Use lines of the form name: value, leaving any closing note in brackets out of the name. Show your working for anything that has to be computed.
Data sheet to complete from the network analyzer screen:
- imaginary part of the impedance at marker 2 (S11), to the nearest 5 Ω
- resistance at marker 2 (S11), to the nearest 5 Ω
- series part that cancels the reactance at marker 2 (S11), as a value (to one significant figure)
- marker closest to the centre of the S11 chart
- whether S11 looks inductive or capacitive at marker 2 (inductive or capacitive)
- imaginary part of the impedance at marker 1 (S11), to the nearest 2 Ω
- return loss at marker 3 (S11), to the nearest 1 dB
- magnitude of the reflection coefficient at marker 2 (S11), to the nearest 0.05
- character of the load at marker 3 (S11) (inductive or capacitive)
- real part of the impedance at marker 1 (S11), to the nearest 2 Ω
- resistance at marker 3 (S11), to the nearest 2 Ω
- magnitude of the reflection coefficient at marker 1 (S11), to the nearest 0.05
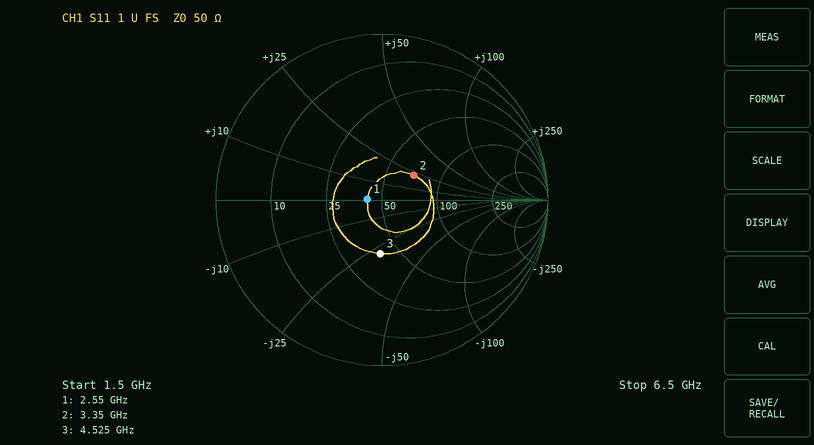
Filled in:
imaginary part of the impedance at marker 2 (S11), to the nearest 5 Ω: +20 Ω
resistance at marker 2 (S11), to the nearest 5 Ω: 70 Ω
series part that cancels the reactance at marker 2 (S11), as a value: C = 1/(2π × 3.35 GHz × 20 Ω) ≈ 2 pF
marker closest to the centre of the S11 chart: marker 1
whether S11 looks inductive or capacitive at marker 2: inductive
imaginary part of the impedance at marker 1 (S11), to the nearest 2 Ω: 0 Ω
return loss at marker 3 (S11), to the nearest 1 dB: 10 dB
magnitude of the reflection coefficient at marker 2 (S11), to the nearest 0.05: 0.25
character of the load at marker 3 (S11): capacitive
real part of the impedance at marker 1 (S11), to the nearest 2 Ω: 42 Ω
resistance at marker 3 (S11), to the nearest 2 Ω: 40 Ω
magnitude of the reflection coefficient at marker 1 (S11), to the nearest 0.05: 0.10
